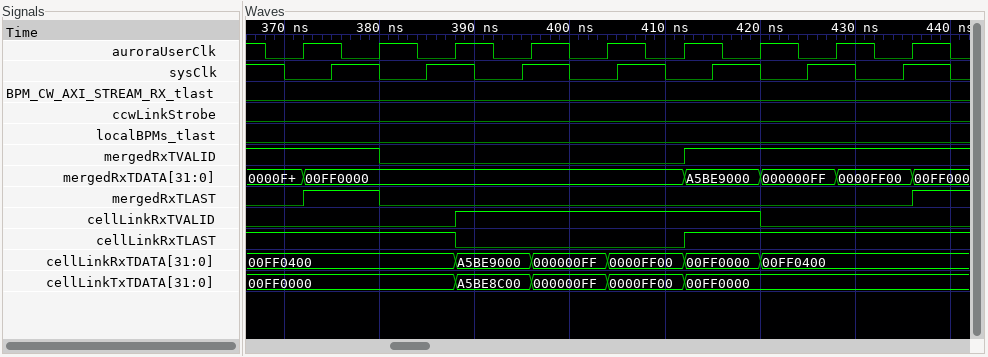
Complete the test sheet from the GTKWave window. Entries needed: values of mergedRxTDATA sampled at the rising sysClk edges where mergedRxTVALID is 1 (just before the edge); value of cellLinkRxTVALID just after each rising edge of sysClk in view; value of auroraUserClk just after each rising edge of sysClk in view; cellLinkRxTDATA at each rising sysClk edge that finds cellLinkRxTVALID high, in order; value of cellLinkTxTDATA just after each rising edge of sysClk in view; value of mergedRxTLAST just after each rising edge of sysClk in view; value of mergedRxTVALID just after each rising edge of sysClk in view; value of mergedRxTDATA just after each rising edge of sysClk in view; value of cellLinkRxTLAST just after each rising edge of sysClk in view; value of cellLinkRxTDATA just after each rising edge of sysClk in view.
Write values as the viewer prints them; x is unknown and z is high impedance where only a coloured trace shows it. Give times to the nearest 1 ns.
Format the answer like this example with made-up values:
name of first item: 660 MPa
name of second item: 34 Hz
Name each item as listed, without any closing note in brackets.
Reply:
values of mergedRxTDATA sampled at the rising sysClk edges where mergedRxTVALID is 1: 00FF0000, A5BE9000, 000000FF, 0000FF00
value of cellLinkRxTVALID just after each rising edge of sysClk in view: 0 0 1 1 1 0 0
value of auroraUserClk just after each rising edge of sysClk in view: 1 0 0 1 1 0 0
cellLinkRxTDATA at each rising sysClk edge that finds cellLinkRxTVALID high, in order: A5BE9000, 0000FF00, 00FF0000
value of cellLinkTxTDATA just after each rising edge of sysClk in view: 00FF0000, 00FF0000, A5BE8C00, 0000FF00, 00FF0000, 00FF0000, 00FF0000
value of mergedRxTLAST just after each rising edge of sysClk in view: 1 0 0 0 0 0 0
value of mergedRxTVALID just after each rising edge of sysClk in view: 1 0 0 0 1 1 1
value of mergedRxTDATA just after each rising edge of sysClk in view: 00FF0000, 00FF0000, 00FF0000, 00FF0000, A5BE9000, 000000FF, 0000FF00
value of cellLinkRxTLAST just after each rising edge of sysClk in view: 1 1 0 0 1 1 1
value of cellLinkRxTDATA just after each rising edge of sysClk in view: 00FF0400, 00FF0400, A5BE9000, 0000FF00, 00FF0000, 00FF0400, 00FF0400
